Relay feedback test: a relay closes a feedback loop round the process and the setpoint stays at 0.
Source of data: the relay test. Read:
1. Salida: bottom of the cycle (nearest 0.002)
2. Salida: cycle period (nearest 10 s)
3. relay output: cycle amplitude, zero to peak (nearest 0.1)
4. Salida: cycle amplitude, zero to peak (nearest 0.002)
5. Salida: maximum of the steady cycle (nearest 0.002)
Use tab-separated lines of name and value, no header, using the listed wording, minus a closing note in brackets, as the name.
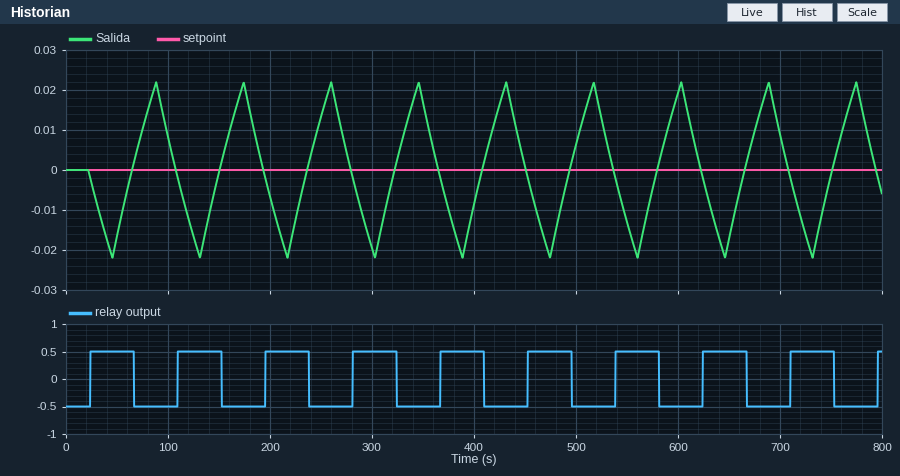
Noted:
Salida: bottom of the cycle	-0.022
Salida: cycle period	90 s
relay output: cycle amplitude, zero to peak	0.5
Salida: cycle amplitude, zero to peak	0.022
Salida: maximum of the steady cycle	0.022
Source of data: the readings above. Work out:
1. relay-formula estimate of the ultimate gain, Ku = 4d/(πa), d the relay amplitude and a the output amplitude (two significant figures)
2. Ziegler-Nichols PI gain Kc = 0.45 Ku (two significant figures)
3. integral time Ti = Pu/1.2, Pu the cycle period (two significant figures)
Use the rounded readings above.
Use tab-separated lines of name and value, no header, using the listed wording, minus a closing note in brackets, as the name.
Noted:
relay-formula estimate of the ultimate gain, Ku = 4d/(πa), d the relay amplitude and a the output amplitude	29
Ziegler-Nichols PI gain Kc = 0.45 Ku	13
integral time Ti = Pu/1.2, Pu the cycle period	75 s
